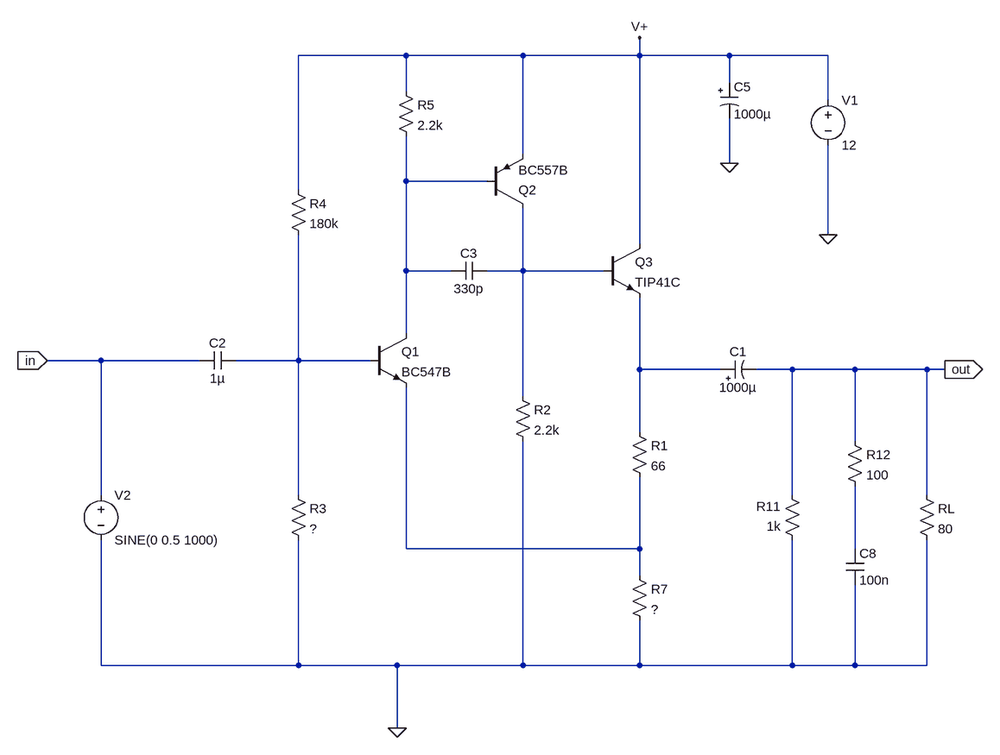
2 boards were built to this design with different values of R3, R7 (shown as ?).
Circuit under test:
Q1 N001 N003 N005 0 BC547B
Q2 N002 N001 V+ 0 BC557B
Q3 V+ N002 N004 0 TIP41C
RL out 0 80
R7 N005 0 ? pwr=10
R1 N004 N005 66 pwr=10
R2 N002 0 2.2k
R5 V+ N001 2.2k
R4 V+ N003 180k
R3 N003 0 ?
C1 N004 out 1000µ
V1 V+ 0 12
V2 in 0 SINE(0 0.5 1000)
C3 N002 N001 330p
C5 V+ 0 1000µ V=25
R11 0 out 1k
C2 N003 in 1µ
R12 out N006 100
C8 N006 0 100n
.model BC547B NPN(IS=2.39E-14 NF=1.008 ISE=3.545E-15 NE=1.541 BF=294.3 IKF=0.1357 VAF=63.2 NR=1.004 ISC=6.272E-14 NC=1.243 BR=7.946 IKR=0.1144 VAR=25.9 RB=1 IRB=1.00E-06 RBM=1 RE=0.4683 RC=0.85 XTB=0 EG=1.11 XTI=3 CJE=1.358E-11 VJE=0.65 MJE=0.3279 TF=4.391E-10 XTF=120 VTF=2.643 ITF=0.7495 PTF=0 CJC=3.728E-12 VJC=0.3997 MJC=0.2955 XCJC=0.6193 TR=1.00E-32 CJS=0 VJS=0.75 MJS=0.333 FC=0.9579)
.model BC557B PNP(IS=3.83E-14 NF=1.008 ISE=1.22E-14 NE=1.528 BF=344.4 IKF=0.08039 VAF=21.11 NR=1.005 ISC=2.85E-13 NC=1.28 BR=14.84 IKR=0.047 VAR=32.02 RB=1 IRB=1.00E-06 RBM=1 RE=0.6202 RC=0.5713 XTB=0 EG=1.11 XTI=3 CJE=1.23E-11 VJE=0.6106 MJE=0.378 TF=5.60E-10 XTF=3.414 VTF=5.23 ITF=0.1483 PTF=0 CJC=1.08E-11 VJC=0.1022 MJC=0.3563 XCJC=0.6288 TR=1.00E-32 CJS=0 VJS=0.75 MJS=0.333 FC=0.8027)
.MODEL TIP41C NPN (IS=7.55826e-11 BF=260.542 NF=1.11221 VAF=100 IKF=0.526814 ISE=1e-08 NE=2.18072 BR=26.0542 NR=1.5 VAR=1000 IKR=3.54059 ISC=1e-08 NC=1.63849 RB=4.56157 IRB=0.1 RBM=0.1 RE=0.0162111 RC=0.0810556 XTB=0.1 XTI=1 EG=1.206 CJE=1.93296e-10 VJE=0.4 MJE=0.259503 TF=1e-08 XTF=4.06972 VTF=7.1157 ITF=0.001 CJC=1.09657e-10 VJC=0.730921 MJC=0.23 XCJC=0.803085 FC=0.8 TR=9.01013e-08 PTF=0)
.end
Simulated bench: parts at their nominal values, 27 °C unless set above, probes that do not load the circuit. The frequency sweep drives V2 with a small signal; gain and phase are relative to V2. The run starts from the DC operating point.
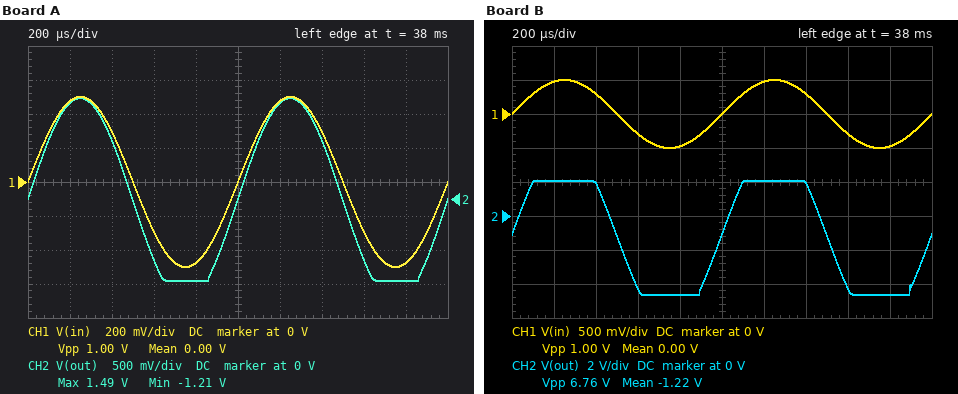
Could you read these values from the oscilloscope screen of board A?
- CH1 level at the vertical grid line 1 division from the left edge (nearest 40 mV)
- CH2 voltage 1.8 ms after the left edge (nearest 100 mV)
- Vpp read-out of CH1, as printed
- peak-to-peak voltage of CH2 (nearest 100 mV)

480 mV
-1.2 V
1.00 V
2.7 V
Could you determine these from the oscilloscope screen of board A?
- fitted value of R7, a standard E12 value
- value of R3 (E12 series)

33 Ω
27 kΩ
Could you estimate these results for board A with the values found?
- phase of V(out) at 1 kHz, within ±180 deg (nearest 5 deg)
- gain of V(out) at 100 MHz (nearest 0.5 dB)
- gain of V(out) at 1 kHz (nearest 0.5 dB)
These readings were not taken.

0 deg
-24.0 dB
9.5 dB
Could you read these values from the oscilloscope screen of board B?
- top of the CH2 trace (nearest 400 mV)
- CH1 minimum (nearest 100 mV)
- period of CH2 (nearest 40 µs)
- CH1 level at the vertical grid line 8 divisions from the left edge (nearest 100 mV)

2.0 V
-500 mV
1.00 ms
-300 mV
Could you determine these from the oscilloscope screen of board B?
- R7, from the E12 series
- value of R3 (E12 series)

6.8 Ω
27 kΩ
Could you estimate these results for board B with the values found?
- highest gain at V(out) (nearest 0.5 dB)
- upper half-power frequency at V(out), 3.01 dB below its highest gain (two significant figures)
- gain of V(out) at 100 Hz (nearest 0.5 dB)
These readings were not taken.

20.5 dB
520 kHz
20.5 dB
